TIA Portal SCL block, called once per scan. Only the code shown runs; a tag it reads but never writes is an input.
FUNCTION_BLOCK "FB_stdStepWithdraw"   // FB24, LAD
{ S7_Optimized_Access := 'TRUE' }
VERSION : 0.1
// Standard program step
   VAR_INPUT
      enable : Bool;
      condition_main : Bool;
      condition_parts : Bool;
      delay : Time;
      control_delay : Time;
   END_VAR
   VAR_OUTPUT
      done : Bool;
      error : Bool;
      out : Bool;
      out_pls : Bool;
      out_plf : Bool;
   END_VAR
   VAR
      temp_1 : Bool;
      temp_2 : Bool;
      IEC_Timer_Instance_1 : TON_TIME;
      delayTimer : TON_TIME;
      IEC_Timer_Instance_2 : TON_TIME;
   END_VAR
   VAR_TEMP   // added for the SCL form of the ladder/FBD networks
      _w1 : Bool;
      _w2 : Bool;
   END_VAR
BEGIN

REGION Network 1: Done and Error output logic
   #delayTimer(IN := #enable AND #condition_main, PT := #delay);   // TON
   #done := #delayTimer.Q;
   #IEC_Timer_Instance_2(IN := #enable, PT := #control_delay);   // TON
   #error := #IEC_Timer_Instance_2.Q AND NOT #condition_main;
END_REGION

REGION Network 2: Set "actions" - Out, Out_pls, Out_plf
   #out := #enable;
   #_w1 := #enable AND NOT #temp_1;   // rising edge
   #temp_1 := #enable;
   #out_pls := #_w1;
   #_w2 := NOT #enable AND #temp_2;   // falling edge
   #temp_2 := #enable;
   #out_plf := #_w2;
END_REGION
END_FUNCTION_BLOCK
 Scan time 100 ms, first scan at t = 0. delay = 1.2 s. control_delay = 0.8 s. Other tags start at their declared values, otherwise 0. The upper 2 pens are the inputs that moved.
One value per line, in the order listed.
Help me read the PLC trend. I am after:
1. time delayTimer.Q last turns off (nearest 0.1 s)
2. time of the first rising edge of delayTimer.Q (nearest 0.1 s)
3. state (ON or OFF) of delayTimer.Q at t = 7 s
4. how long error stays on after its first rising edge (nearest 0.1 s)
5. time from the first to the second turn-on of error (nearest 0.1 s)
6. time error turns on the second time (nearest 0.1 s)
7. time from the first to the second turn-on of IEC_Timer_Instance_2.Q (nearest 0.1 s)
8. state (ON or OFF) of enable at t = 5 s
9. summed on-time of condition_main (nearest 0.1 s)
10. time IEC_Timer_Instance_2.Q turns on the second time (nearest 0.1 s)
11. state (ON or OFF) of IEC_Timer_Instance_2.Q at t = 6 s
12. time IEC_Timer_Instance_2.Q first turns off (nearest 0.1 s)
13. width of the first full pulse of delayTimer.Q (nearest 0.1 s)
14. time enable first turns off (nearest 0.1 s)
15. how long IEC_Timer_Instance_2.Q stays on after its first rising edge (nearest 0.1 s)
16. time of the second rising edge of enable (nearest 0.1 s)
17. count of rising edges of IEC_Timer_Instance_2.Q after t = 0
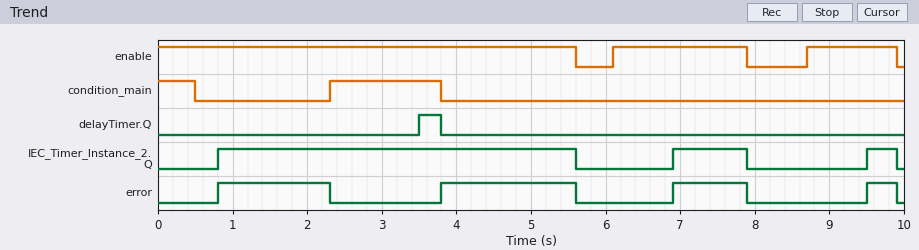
3.8 s
3.5 s
OFF
1.5 s
3.0 s
3.8 s
6.1 s
ON
2.0 s
6.9 s
OFF
5.6 s
0.3 s
5.6 s
4.8 s
8.7 s
3
